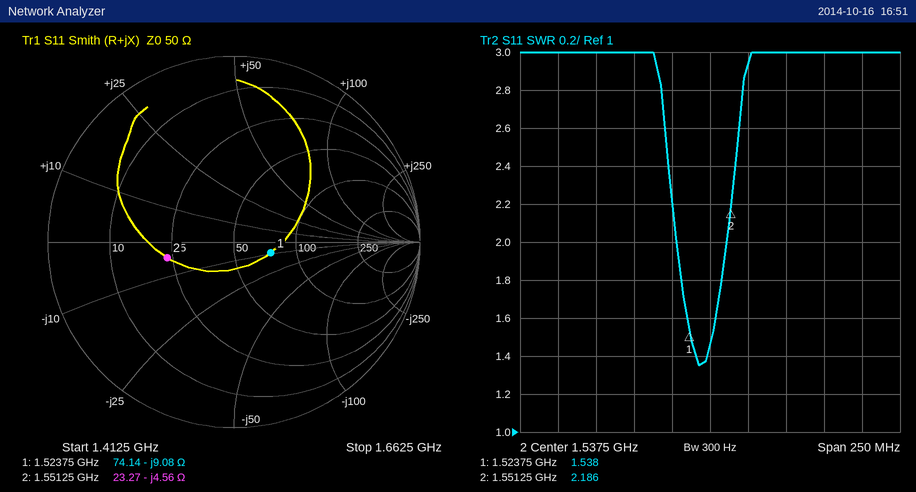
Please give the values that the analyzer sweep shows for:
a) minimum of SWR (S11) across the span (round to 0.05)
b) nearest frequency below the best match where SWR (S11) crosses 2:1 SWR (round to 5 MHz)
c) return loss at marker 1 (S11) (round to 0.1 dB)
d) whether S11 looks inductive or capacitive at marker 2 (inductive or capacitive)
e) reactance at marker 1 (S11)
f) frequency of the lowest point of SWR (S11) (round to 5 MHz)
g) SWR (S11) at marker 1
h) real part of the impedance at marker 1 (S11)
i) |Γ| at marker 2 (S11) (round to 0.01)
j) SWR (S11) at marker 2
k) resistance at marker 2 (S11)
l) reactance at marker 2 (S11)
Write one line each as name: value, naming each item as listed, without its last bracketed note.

minimum of SWR (S11) across the span: 1.35
nearest frequency below the best match where SWR (S11) crosses 2:1 SWR: 1.515 GHz
return loss at marker 1 (S11): 13.7 dB
whether S11 looks inductive or capacitive at marker 2: capacitive
reactance at marker 1: -9.08 Ω
frequency of the lowest point of SWR (S11): 1.530 GHz
SWR (S11) at marker 1: 1.538
real part of the impedance at marker 1: 74.14 Ω
|Γ| at marker 2 (S11): 0.37
SWR (S11) at marker 2: 2.186
resistance at marker 2: 23.27 Ω
reactance at marker 2: -4.56 Ω
